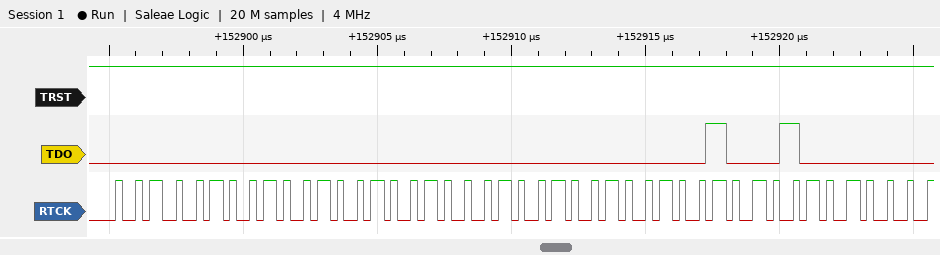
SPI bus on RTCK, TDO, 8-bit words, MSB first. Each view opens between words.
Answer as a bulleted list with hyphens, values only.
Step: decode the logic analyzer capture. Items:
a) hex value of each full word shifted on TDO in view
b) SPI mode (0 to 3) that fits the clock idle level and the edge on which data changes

- 00, 00, 00, 00, 44
- 0
